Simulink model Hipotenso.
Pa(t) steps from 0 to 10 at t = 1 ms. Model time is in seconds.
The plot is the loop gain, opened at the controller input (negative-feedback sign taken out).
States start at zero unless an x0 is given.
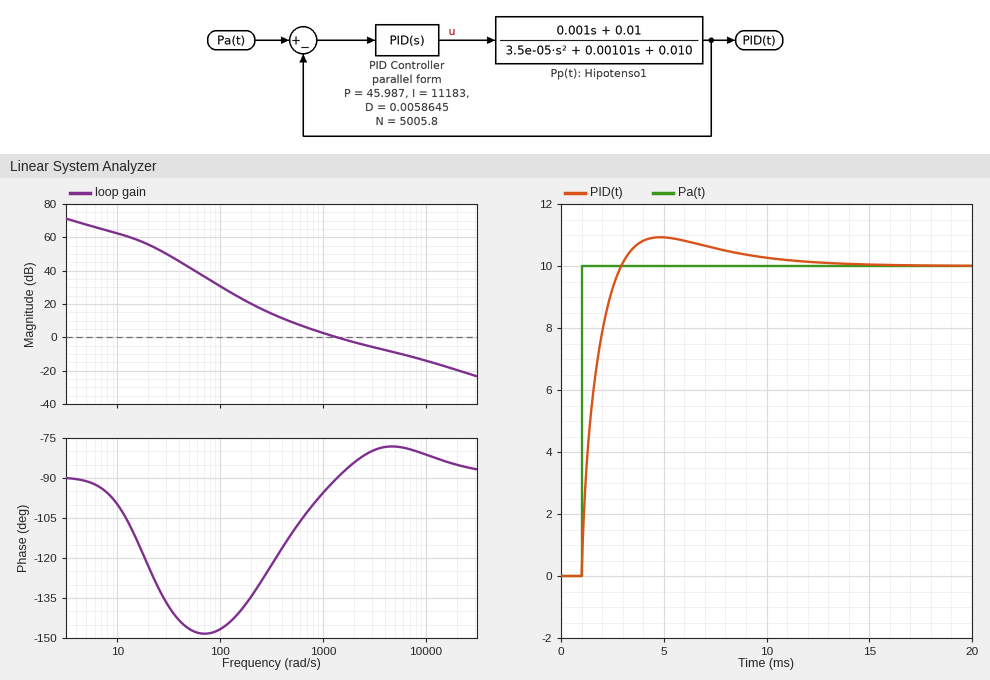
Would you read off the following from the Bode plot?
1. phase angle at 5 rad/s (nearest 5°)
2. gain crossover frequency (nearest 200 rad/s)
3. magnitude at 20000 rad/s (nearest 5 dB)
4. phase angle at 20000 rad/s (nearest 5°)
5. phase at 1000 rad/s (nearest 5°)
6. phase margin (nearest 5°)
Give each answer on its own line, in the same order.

-90°
1400 rad/s
-20 dB
-85°
-95°
90°
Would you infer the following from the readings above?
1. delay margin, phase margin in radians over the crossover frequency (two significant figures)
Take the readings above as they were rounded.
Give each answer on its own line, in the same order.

0.0011 s
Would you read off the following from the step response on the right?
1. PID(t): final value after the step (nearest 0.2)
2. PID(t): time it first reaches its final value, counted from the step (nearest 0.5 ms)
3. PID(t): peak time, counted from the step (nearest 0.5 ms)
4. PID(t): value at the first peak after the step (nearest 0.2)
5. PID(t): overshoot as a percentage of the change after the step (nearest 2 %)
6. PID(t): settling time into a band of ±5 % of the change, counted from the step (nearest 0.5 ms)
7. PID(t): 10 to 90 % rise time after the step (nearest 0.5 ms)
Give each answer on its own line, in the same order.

10.0
2.0 ms
4.0 ms
11.0
10 %
7.0 ms
1.5 ms
